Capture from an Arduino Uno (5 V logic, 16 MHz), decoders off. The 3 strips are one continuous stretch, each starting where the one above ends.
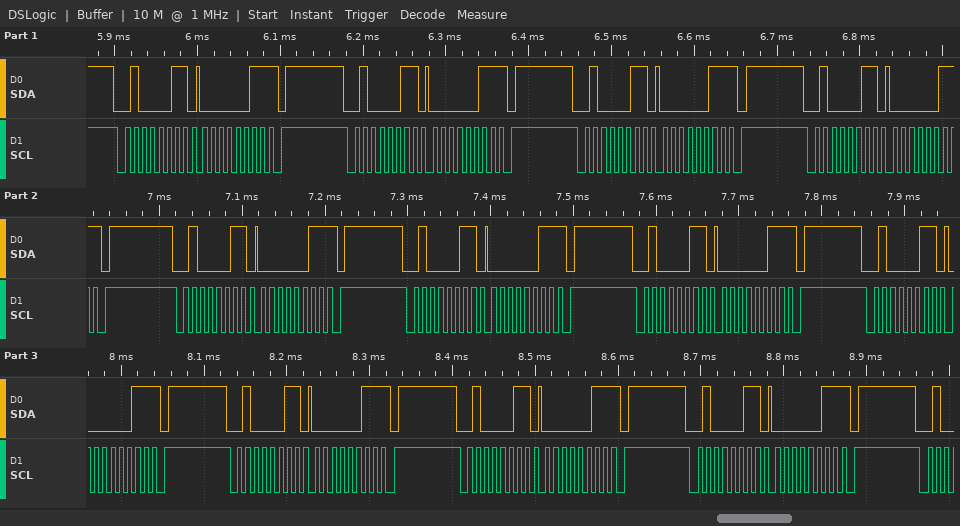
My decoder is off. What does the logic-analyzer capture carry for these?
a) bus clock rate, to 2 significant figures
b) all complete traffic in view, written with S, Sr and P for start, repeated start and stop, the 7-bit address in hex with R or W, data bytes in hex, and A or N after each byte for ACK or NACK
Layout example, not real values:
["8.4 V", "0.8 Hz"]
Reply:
["100 kHz", "S 21R A 03 N P S 21R A 03 N P S 21R A 03 N P S 21R A 03 N P S 21R A 03 N P S 21R A 03 N P S 21R A 03 N P S 21R A 03 N P S 21R A 03 N P S 21R A 03 N P S 21R A 03 N P"]
